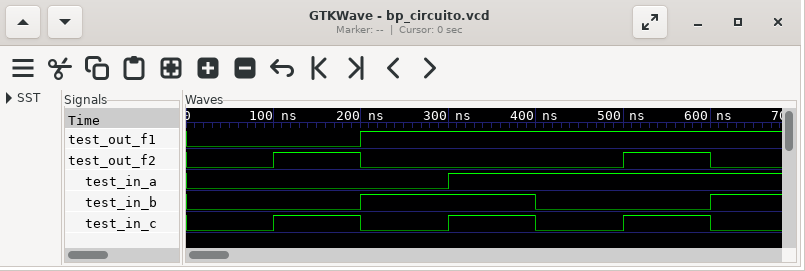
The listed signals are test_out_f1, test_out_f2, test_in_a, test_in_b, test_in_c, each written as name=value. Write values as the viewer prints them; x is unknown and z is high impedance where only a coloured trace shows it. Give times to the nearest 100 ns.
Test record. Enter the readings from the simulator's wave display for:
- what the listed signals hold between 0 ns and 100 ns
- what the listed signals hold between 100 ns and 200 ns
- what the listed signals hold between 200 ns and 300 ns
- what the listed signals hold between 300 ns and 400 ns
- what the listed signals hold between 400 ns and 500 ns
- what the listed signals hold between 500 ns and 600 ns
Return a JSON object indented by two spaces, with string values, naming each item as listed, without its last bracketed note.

{
  "what the listed signals hold between 0 ns and 100 ns": "test_out_f1=0, test_out_f2=0, test_in_a=0, test_in_b=0, test_in_c=0",
  "what the listed signals hold between 100 ns and 200 ns": "test_out_f1=0, test_out_f2=1, test_in_a=0, test_in_b=0, test_in_c=1",
  "what the listed signals hold between 200 ns and 300 ns": "test_out_f1=1, test_out_f2=0, test_in_a=0, test_in_b=1, test_in_c=0",
  "what the listed signals hold between 300 ns and 400 ns": "test_out_f1=1, test_out_f2=0, test_in_a=1, test_in_b=1, test_in_c=1",
  "what the listed signals hold between 400 ns and 500 ns": "test_out_f1=1, test_out_f2=0, test_in_a=1, test_in_b=0, test_in_c=0",
  "what the listed signals hold between 500 ns and 600 ns": "test_out_f1=1, test_out_f2=1, test_in_a=1, test_in_b=0, test_in_c=1"
}
